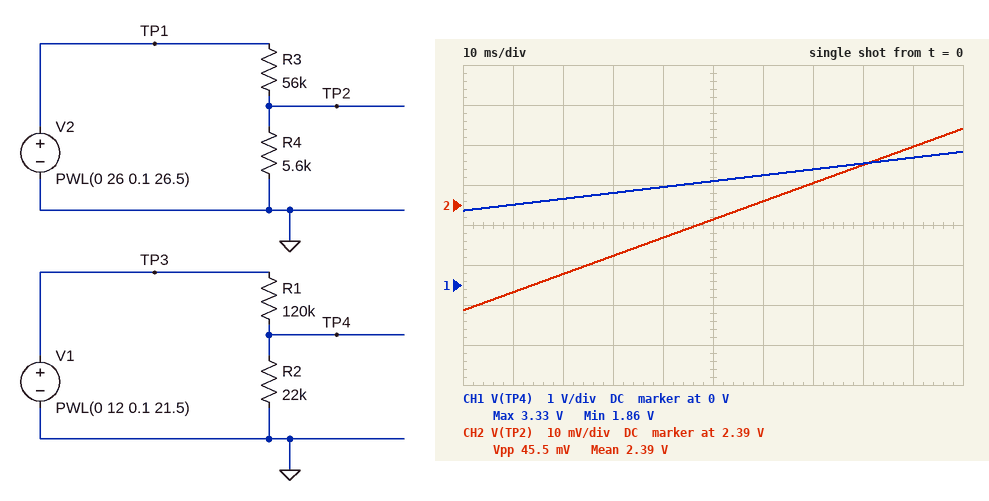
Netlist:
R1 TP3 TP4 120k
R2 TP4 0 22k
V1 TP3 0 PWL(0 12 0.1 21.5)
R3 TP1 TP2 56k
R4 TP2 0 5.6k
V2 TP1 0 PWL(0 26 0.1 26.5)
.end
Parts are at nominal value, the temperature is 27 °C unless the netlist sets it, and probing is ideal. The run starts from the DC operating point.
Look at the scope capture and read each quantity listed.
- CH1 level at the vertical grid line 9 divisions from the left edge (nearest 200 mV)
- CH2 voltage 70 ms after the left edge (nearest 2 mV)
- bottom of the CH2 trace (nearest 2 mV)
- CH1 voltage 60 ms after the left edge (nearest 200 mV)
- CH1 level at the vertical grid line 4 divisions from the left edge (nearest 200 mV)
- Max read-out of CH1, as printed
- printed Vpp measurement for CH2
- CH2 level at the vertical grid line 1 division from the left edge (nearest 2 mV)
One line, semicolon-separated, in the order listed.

3.2 V; 2.396 V; 2.364 V; 2.8 V; 2.4 V; 3.33 V; 45.5 mV; 2.368 V
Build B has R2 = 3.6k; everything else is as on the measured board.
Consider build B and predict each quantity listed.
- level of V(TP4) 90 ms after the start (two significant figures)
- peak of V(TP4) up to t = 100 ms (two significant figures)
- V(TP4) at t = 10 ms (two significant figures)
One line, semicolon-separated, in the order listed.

600 mV; 630 mV; 380 mV
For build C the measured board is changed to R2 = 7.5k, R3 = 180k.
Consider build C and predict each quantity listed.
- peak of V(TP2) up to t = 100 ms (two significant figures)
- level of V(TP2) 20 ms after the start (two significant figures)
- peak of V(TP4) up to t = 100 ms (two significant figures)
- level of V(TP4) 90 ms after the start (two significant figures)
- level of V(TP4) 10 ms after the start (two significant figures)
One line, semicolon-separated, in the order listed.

800 mV; 790 mV; 1.3 V; 1.2 V; 760 mV
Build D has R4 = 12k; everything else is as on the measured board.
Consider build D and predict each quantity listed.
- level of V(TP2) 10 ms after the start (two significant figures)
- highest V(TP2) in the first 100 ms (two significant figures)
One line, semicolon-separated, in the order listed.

4.6 V; 4.7 V
